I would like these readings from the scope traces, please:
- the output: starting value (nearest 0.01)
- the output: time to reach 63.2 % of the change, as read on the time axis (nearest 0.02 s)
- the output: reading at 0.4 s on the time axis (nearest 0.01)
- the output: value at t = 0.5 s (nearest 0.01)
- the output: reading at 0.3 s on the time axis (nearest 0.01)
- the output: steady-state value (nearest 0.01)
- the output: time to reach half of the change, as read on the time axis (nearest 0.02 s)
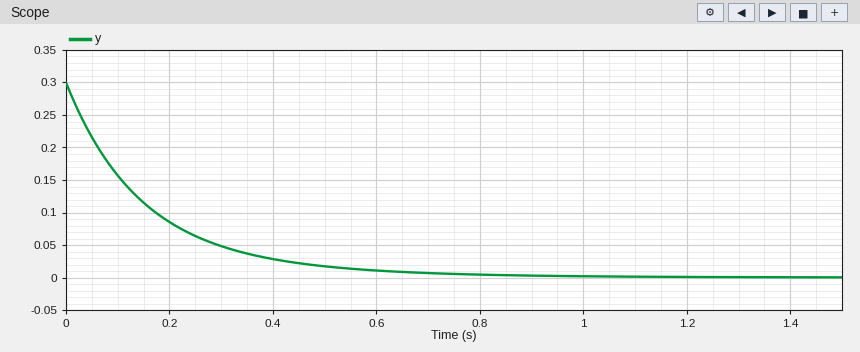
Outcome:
0.30
0.16 s
0.03
0.02
0.05
0.00
0.10 s
